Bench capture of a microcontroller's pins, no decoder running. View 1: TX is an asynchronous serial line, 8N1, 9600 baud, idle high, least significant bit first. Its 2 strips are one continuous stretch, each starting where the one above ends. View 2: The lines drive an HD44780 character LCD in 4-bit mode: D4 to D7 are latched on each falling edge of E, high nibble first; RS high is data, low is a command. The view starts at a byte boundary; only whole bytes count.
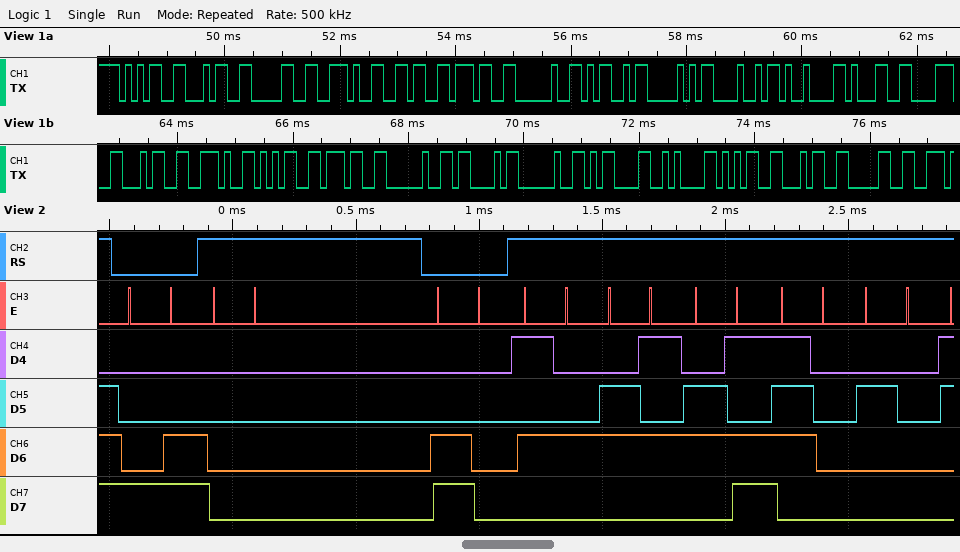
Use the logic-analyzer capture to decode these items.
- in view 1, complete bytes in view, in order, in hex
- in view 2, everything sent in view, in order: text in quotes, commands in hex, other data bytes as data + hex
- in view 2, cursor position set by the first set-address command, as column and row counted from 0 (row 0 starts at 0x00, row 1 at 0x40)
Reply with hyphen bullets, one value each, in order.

- 35 34 30 2E 36 37 20 4D 50 48 09 31 38 34 2E 35 37 20 43 20 0D 0A 35 34 30
- 0x8C data 00 0xC0 "Temp "
- column 12, row 0
